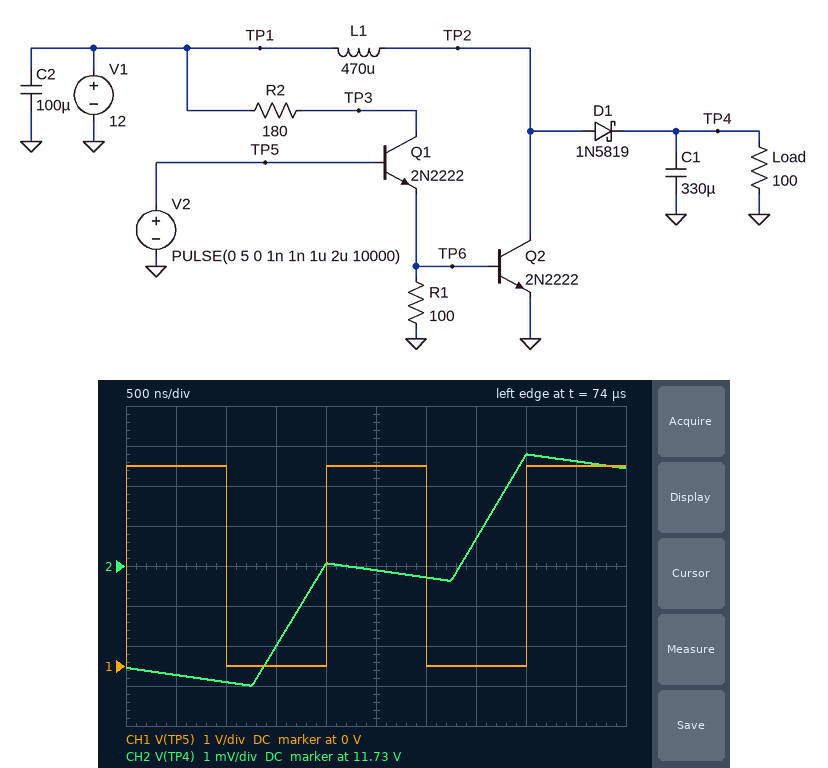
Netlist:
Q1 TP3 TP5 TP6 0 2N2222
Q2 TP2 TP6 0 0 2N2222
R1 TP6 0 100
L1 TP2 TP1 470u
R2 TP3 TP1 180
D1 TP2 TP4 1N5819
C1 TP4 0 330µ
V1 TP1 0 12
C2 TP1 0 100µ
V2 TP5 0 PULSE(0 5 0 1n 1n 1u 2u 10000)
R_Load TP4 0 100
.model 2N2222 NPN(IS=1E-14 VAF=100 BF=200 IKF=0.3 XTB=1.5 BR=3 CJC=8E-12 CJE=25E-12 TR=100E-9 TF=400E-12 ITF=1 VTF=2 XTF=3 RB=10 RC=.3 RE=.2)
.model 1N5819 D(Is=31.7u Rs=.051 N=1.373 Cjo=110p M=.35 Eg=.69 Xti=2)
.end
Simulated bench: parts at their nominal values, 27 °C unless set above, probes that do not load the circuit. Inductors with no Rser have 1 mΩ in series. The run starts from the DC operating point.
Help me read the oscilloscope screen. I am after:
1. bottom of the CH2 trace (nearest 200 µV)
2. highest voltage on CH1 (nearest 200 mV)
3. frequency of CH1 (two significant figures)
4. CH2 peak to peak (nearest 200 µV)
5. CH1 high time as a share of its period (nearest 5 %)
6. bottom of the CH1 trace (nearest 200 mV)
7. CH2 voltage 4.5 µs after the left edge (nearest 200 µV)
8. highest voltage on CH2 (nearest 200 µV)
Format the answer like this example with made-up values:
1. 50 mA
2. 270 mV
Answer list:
1. 11.7300 V
2. 5.0 V
3. 500 kHz
4. 5.8 mV
5. 50 %
6. 0 V
7. 11.7356 V
8. 11.7358 V
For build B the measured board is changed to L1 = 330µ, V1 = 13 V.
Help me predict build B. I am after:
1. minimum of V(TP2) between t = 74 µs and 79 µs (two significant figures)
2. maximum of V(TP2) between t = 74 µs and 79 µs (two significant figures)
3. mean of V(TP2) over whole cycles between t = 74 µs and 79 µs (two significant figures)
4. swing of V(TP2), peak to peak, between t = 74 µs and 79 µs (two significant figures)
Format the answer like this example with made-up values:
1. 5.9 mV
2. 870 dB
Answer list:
1. 1.1 V
2. 13 V
3. 6.6 V
4. 12 V
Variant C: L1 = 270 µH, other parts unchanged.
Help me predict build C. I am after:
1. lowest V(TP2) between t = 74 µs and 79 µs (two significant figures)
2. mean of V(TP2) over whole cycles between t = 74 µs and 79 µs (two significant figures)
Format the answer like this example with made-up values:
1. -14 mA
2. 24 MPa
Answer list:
1. 1.2 V
2. 6.4 V
